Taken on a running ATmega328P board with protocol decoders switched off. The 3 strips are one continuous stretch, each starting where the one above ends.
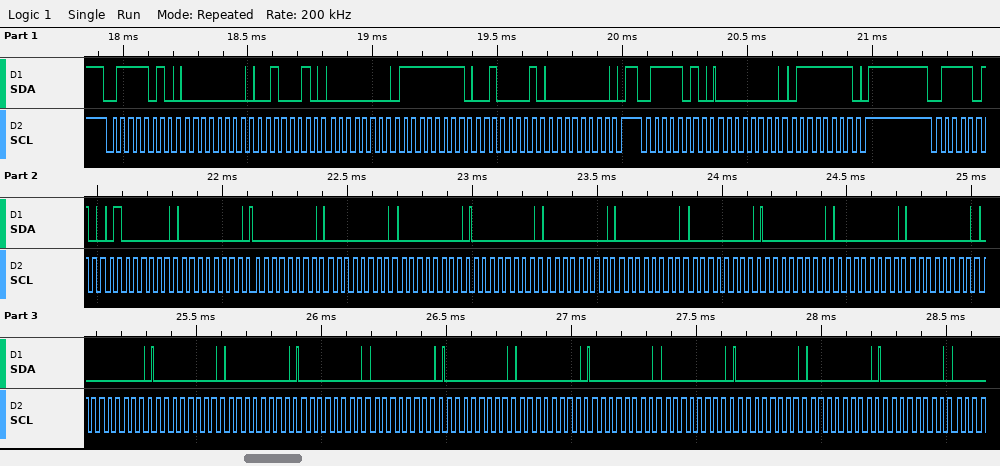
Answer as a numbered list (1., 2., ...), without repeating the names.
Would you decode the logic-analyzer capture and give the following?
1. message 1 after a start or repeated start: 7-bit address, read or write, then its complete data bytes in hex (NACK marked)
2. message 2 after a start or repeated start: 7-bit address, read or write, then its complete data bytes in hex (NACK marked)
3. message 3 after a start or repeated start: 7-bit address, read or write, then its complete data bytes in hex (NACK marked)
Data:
1. 0x3D write: 00 22 00 FF 21 00
2. 0x3D write: 00 7F
3. 0x3D write: 40 00 00 00 00 00 00 00 00 00 00 00 00 00 00 00 00 00 00 00 00 00 00 00
